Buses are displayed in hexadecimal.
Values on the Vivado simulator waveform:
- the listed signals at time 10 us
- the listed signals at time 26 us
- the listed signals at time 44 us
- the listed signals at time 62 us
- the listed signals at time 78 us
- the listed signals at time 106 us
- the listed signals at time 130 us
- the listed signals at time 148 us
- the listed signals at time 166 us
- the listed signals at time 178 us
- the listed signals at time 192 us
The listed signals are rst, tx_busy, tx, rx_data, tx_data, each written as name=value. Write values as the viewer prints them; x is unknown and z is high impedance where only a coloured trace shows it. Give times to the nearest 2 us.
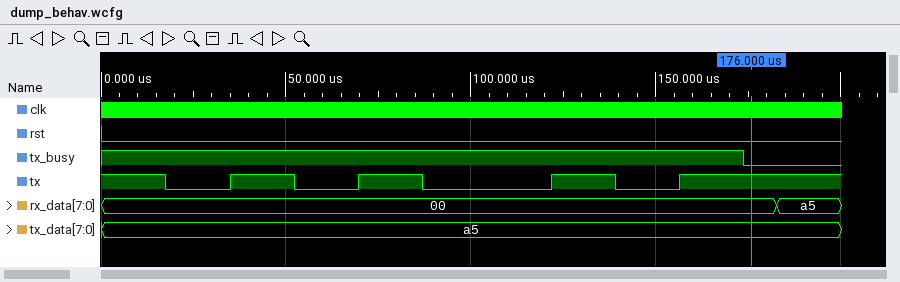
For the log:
rst=0, tx_busy=1, tx=1, rx_data=00, tx_data=a5
rst=0, tx_busy=1, tx=0, rx_data=00, tx_data=a5
rst=0, tx_busy=1, tx=1, rx_data=00, tx_data=a5
rst=0, tx_busy=1, tx=0, rx_data=00, tx_data=a5
rst=0, tx_busy=1, tx=1, rx_data=00, tx_data=a5
rst=0, tx_busy=1, tx=0, rx_data=00, tx_data=a5
rst=0, tx_busy=1, tx=1, rx_data=00, tx_data=a5
rst=0, tx_busy=1, tx=0, rx_data=00, tx_data=a5
rst=0, tx_busy=1, tx=1, rx_data=00, tx_data=a5
rst=0, tx_busy=0, tx=1, rx_data=00, tx_data=a5
rst=0, tx_busy=0, tx=1, rx_data=a5, tx_data=a5
